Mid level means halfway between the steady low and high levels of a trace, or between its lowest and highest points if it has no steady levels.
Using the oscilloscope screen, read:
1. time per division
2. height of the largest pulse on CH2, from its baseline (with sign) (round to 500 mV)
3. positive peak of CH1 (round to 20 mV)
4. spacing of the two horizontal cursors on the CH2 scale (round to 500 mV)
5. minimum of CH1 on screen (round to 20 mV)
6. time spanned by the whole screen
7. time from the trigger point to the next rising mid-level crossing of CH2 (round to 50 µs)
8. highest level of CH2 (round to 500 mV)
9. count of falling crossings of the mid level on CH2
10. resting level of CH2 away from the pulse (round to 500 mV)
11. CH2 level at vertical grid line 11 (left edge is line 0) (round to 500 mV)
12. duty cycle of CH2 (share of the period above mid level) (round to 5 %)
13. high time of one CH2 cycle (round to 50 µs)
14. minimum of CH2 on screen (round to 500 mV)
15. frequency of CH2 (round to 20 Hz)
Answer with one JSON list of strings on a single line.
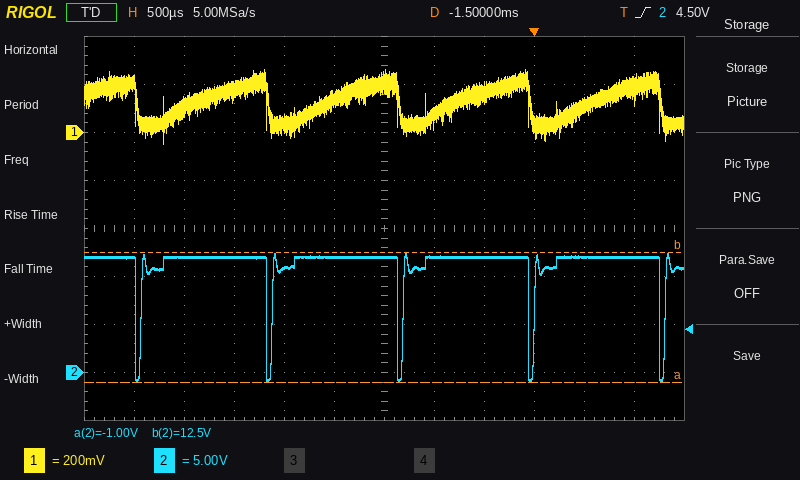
["500 µs", "-13.0 V", "260 mV", "13.5 V", "-40 mV", "6 ms", "1.30 ms", "12.5 V", "5", "12.0 V", "12.0 V", "95 %", "1.25 ms", "-1.0 V", "760 Hz"]
